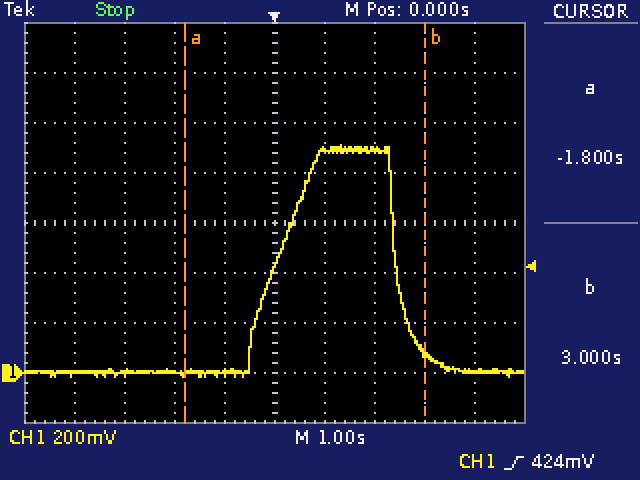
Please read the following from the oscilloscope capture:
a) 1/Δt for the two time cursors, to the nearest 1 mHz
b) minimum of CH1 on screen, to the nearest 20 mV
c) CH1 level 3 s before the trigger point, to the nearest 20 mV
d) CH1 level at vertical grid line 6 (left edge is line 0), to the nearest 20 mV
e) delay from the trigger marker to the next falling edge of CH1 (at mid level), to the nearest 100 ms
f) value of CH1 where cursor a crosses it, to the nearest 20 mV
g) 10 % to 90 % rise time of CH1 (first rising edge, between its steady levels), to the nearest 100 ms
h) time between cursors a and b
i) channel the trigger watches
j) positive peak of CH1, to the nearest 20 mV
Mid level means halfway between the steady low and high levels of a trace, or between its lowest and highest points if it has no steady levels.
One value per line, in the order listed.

208 mHz
-20 mV
0 mV
900 mV
2.4 s
0 mV
1.2 s
4.8 s
CH1
920 mV
